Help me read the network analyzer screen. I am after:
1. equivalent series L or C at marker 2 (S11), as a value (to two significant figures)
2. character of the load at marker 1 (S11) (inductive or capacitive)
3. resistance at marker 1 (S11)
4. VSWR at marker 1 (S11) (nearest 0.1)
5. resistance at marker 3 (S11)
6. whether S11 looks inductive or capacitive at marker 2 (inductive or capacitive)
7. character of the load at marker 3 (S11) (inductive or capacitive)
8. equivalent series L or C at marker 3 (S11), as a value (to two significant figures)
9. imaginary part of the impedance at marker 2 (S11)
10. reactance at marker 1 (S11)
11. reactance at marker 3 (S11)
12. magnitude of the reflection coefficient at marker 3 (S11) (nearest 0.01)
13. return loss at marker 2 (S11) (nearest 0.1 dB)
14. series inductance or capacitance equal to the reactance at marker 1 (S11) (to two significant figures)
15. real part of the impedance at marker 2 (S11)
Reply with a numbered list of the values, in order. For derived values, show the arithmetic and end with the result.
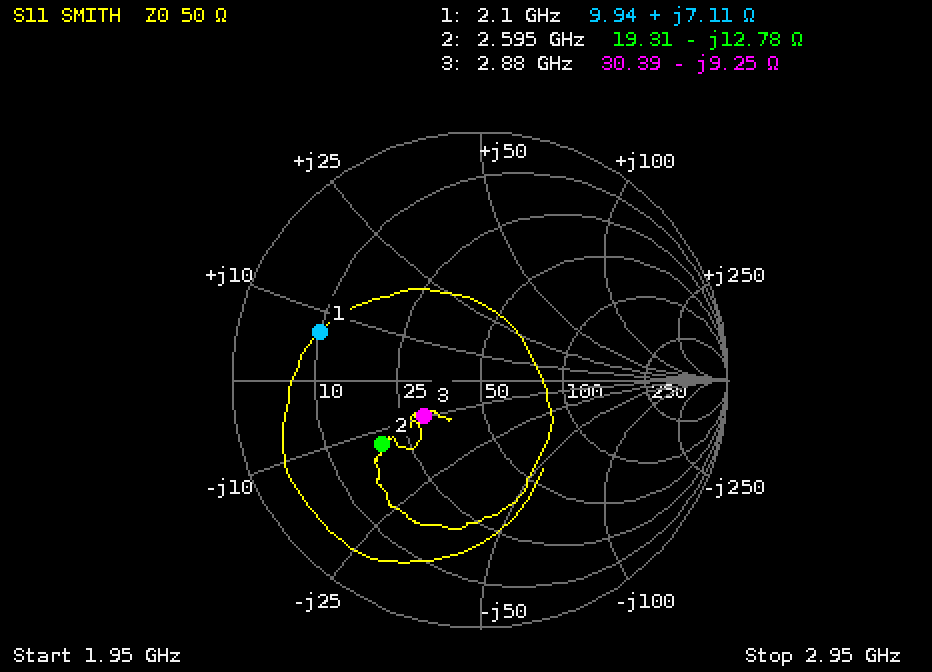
1. C = 1/(2π × 2.595 GHz × 12.78 Ω) ≈ 4.8 pF
2. inductive
3. 9.94 Ω
4. 5.1
5. 30.39 Ω
6. capacitive
7. capacitive
8. C = 1/(2π × 2.88 GHz × 9.25 Ω) ≈ 6.0 pF
9. -12.78 Ω
10. +7.11 Ω
11. -9.25 Ω
12. 0.27
13. 6.5 dB
14. L = 7.11 Ω/(2π × 2.1 GHz) ≈ 539 pH, so 540 pH to two significant figures
15. 19.31 Ω
